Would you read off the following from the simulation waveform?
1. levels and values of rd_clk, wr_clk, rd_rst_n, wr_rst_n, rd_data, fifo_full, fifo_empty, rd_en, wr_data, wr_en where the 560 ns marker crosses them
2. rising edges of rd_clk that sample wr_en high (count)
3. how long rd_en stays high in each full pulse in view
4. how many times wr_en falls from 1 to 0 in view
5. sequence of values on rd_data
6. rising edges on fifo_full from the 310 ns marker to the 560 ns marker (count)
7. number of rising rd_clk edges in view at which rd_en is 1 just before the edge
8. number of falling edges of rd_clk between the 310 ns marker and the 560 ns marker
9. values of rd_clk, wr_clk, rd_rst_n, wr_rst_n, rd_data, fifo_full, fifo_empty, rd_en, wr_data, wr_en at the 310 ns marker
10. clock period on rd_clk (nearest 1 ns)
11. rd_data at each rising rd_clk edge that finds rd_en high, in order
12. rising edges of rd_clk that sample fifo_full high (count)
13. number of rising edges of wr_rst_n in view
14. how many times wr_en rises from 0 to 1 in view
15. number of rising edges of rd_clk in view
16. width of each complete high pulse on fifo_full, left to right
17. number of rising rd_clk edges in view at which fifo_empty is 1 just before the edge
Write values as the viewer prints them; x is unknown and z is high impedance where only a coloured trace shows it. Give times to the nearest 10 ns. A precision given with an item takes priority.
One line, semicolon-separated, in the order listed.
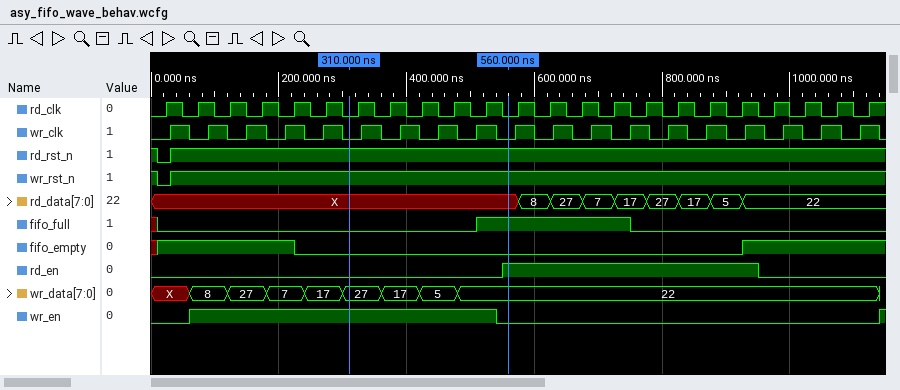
rd_clk=0, wr_clk=0, rd_rst_n=1, wr_rst_n=1, rd_data=X, fifo_full=1, fifo_empty=0, rd_en=1, wr_data=22, wr_en=0; 10; 400 ns; 1; X, 8, 27, 7, 17, 27, 17, 5, 22; 1; 8; 5; rd_clk=0, wr_clk=0, rd_rst_n=1, wr_rst_n=1, rd_data=X, fifo_full=0, fifo_empty=0, rd_en=0, wr_data=27, wr_en=1; 50 ns; X, 8, 27, 7, 17, 27, 17, 5; 5; 1; 2; 23; 240 ns; 9
